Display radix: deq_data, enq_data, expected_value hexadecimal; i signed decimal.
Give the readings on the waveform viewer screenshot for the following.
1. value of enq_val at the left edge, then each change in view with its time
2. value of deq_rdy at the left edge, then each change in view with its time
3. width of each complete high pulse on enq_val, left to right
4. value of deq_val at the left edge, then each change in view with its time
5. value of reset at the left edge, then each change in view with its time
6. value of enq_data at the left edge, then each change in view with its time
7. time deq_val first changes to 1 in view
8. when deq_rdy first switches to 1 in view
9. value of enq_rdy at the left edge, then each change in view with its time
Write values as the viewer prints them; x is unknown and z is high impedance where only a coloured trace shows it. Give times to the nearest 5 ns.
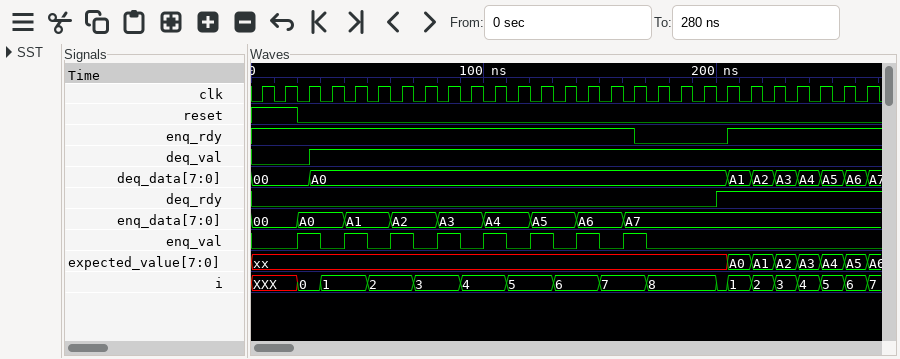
0, 1 at 20 ns, 0 at 30 ns, 1 at 40 ns, 0 at 50 ns, 1 at 60 ns, 0 at 70 ns, 1 at 80 ns, 0 at 90 ns, 1 at 100 ns, 0 at 110 ns, 1 at 120 ns, 0 at 130 ns, 1 at 140 ns, 0 at 150 ns, 1 at 160 ns, 0 at 170 ns
0, 1 at 200 ns
10 ns, 10 ns, 10 ns, 10 ns, 10 ns, 10 ns, 10 ns, 10 ns
0, 1 at 25 ns
1, 0 at 20 ns
00, A0 at 20 ns, A1 at 40 ns, A2 at 60 ns, A3 at 80 ns, A4 at 100 ns, A5 at 120 ns, A6 at 140 ns, A7 at 160 ns
25 ns
200 ns
1, 0 at 165 ns, 1 at 205 ns
